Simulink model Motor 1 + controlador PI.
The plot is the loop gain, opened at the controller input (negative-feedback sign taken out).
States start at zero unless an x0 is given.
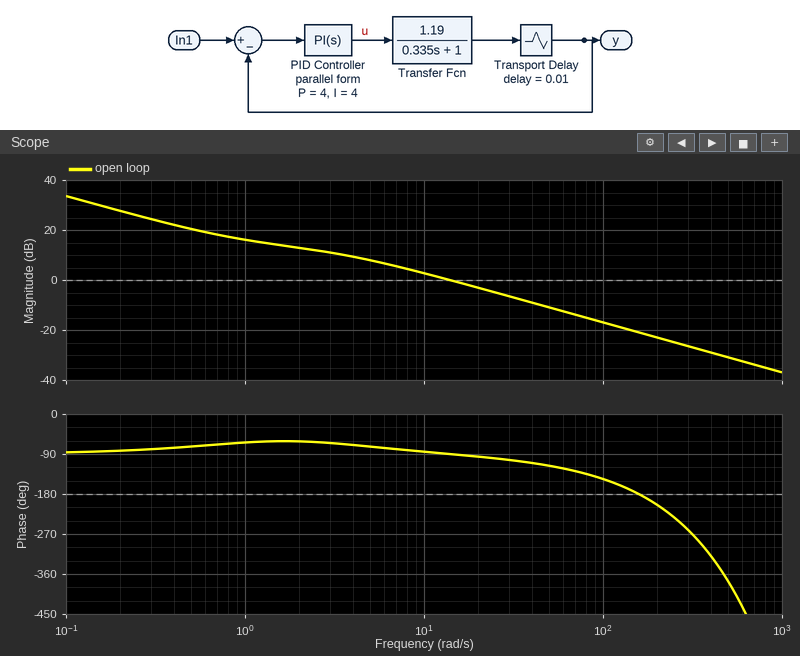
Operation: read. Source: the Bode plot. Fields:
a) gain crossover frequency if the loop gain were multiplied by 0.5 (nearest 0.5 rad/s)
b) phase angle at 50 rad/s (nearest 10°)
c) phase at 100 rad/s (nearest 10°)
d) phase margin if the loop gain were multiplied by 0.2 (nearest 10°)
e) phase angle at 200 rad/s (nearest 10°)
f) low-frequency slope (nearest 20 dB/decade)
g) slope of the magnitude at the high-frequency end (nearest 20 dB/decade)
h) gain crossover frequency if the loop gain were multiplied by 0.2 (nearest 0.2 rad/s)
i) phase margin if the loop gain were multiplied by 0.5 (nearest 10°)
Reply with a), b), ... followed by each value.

a) 6.5 rad/s
b) -120°
c) -150°
d) 120°
e) -200°
f) -20 dB/decade
g) -20 dB/decade
h) 1.6 rad/s
i) 100°
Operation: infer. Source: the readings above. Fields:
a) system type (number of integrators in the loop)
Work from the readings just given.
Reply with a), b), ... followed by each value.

a) 1
